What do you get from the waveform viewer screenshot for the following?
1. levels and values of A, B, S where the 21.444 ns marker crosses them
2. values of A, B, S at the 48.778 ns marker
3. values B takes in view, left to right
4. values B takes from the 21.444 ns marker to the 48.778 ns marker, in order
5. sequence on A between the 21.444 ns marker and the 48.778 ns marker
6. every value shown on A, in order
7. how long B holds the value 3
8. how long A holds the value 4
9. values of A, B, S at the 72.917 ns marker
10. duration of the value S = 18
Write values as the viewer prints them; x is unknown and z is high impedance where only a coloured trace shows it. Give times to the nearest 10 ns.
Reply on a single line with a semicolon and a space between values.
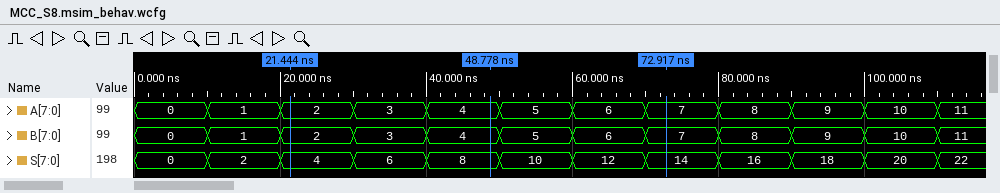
A=2, B=2, S=4; A=4, B=4, S=8; 0, 1, 2, 3, 4, 5, 6, 7, 8, 9, 10, 11; 2, 3, 4; 2, 3, 4; 0, 1, 2, 3, 4, 5, 6, 7, 8, 9, 10, 11; 10 ns; 10 ns; A=7, B=7, S=14; 10 ns
